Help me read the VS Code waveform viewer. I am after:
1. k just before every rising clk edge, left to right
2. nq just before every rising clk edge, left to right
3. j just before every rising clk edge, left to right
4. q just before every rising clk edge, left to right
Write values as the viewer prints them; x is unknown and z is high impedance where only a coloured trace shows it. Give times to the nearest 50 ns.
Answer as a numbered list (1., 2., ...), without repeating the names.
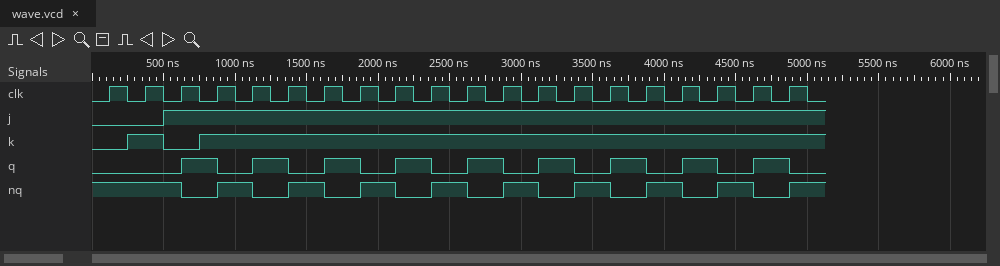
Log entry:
1. 0 1 0 1 1 1 1 1 1 1 1 1 1 1 1 1 1 1 1 1
2. 1 1 1 0 1 0 1 0 1 0 1 0 1 0 1 0 1 0 1 0
3. 0 0 1 1 1 1 1 1 1 1 1 1 1 1 1 1 1 1 1 1
4. 0 0 0 1 0 1 0 1 0 1 0 1 0 1 0 1 0 1 0 1
